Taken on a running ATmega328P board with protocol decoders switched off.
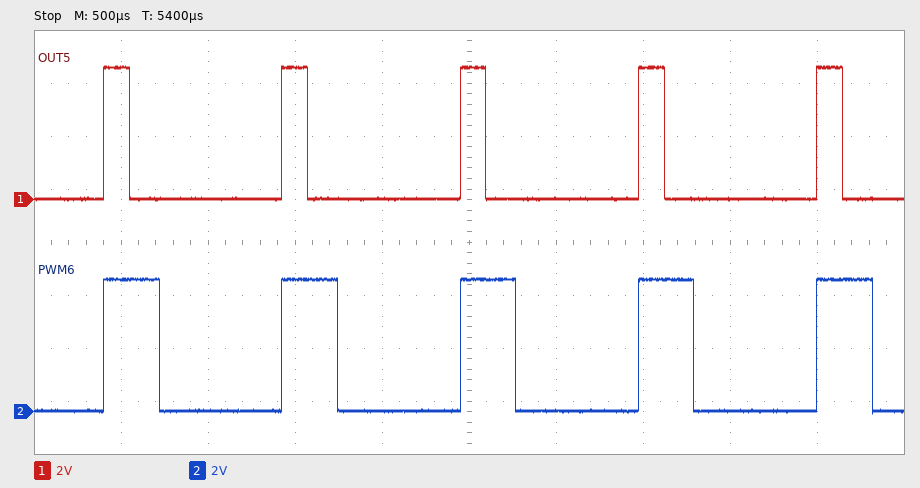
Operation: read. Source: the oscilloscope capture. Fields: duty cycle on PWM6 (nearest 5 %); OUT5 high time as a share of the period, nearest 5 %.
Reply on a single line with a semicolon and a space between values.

30 %; 15 %
